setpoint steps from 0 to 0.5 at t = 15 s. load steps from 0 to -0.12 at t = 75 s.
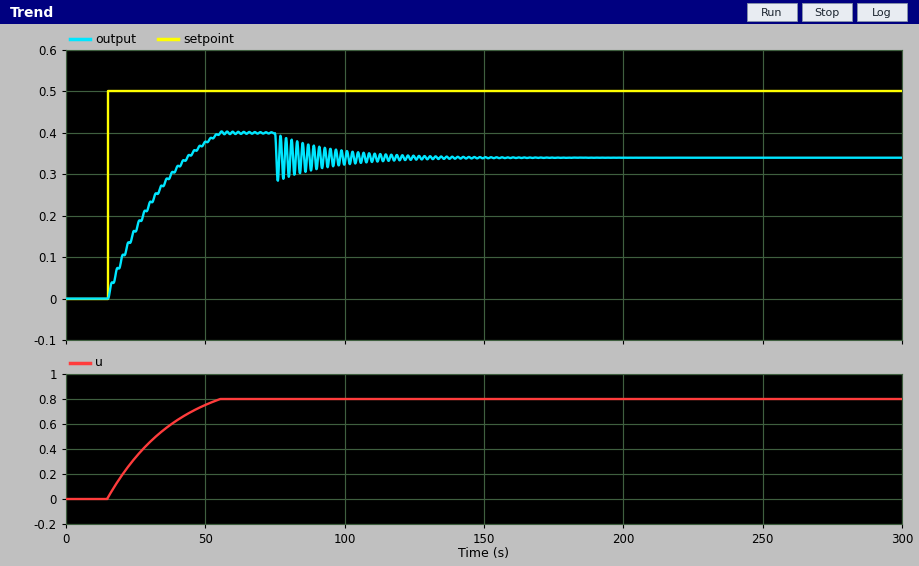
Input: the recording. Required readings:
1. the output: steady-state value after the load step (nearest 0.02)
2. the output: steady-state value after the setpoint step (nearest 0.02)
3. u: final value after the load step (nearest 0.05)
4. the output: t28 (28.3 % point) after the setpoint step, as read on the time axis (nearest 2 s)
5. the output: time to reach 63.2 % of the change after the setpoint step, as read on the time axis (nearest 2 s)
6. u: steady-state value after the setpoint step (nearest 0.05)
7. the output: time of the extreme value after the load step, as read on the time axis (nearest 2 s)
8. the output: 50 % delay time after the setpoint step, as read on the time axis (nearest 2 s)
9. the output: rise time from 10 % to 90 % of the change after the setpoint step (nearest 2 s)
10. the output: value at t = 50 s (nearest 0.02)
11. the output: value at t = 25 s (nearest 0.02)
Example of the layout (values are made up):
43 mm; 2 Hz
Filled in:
0.34; 0.40; 0.80; 22 s; 32 s; 0.80; 76 s; 28 s; 30 s; 0.38; 0.16
